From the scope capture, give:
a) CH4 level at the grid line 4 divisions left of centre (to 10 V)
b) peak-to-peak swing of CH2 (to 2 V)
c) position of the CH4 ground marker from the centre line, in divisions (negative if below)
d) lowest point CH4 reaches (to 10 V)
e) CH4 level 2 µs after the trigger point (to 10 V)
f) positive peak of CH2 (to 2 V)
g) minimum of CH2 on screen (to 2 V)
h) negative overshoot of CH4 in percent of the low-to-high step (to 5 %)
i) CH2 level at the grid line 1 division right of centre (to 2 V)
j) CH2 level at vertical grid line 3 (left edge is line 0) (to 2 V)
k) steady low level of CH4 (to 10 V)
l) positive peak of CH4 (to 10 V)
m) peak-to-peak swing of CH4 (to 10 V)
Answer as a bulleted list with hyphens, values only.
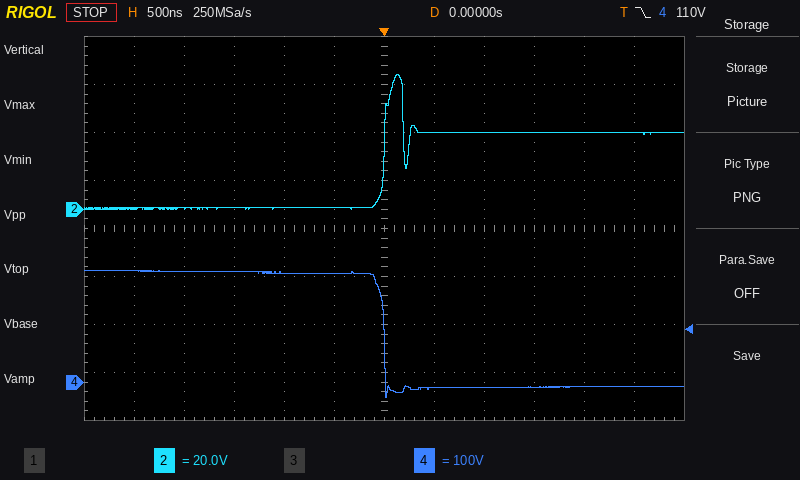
- 230 V
- 56 V
- -3.2 div
- -30 V
- -10 V
- 56 V
- 0 V
- 10 %
- 32 V
- 0 V
- -10 V
- 230 V
- 260 V
